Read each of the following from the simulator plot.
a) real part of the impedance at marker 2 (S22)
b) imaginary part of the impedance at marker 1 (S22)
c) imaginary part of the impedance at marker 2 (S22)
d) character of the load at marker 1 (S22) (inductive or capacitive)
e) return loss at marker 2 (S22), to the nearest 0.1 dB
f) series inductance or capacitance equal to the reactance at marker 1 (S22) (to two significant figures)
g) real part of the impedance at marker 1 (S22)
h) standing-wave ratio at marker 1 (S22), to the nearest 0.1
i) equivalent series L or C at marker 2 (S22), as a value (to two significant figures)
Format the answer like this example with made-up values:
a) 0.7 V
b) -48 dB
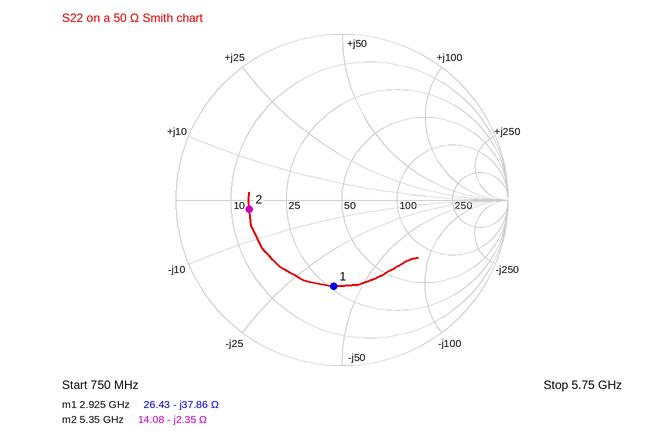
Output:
a) 14.08 Ω
b) -37.86 Ω
c) -2.35 Ω
d) capacitive
e) 5.0 dB
f) 1.4 pF
g) 26.43 Ω
h) 3.2
i) 13 pF
